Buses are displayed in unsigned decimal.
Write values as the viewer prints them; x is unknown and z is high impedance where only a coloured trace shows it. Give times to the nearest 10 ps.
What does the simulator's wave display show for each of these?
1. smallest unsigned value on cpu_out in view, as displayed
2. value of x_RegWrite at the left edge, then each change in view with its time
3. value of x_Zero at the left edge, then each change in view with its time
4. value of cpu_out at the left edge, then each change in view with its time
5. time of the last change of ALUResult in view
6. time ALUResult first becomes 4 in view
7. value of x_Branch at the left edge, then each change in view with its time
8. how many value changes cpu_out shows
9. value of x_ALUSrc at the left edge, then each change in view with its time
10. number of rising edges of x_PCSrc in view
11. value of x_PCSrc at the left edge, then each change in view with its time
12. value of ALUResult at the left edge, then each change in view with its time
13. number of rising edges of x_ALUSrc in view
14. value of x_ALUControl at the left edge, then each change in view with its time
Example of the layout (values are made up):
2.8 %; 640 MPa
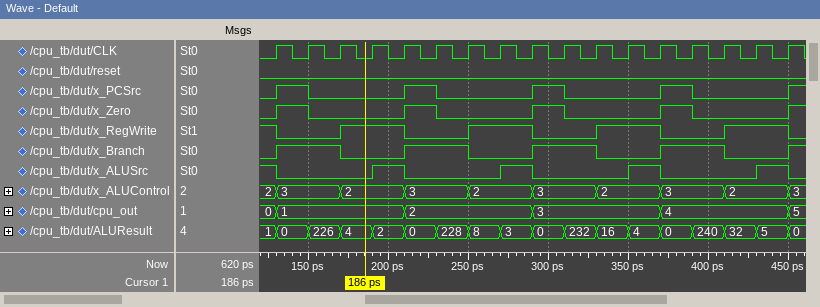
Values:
0; 1, 0 at 130 ps, 1 at 170 ps, 0 at 210 ps, 1 at 250 ps, 0 at 290 ps, 1 at 330 ps, 0 at 370 ps, 1 at 410 ps, 0 at 450 ps; 0, 1 at 130 ps, 0 at 150 ps, 1 at 210 ps, 0 at 230 ps, 1 at 290 ps, 0 at 310 ps, 1 at 370 ps, 0 at 390 ps, 1 at 450 ps; 0, 1 at 130 ps, 2 at 210 ps, 3 at 290 ps, 4 at 370 ps, 5 at 450 ps; 450 ps; 170 ps; 0, 1 at 130 ps, 0 at 170 ps, 1 at 210 ps, 0 at 250 ps, 1 at 290 ps, 0 at 330 ps, 1 at 370 ps, 0 at 410 ps, 1 at 450 ps; 5; 1, 0 at 130 ps, 1 at 190 ps, 0 at 210 ps, 1 at 270 ps, 0 at 290 ps, 1 at 350 ps, 0 at 370 ps, 1 at 430 ps, 0 at 450 ps; 5; 0, 1 at 130 ps, 0 at 150 ps, 1 at 210 ps, 0 at 230 ps, 1 at 290 ps, 0 at 310 ps, 1 at 370 ps, 0 at 390 ps, 1 at 450 ps; 1, 0 at 130 ps, 226 at 150 ps, 4 at 170 ps, 2 at 190 ps, 0 at 210 ps, 228 at 230 ps, 8 at 250 ps, 3 at 270 ps, 0 at 290 ps, 232 at 310 ps, 16 at 330 ps, 4 at 350 ps, 0 at 370 ps, 240 at 390 ps, 32 at 410 ps, 5 at 430 ps, 0 at 450 ps; 4; 2, 3 at 130 ps, 2 at 170 ps, 3 at 210 ps, 2 at 250 ps, 3 at 290 ps, 2 at 330 ps, 3 at 370 ps, 2 at 410 ps, 3 at 450 ps
